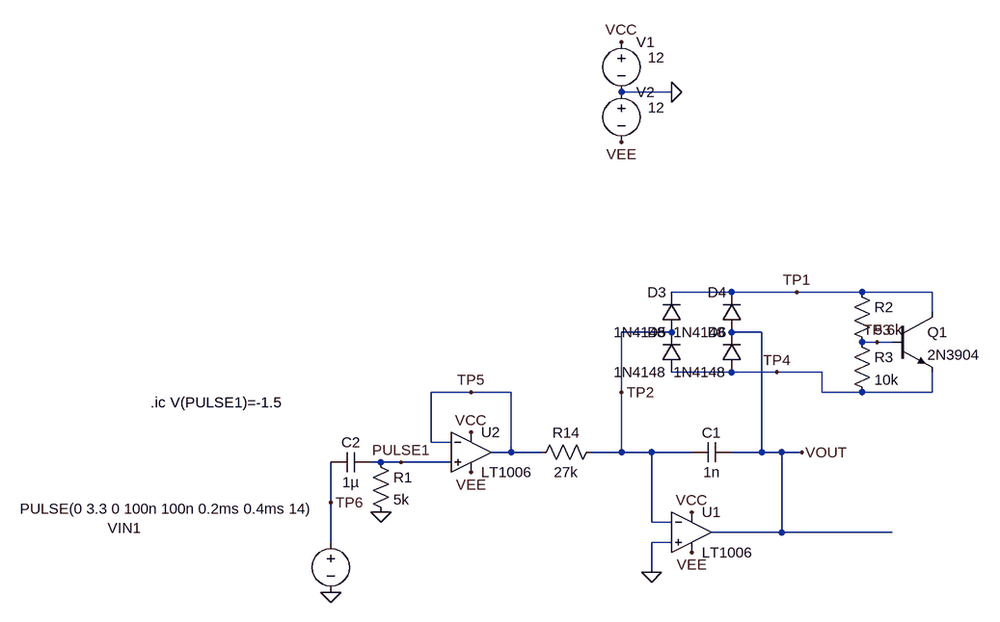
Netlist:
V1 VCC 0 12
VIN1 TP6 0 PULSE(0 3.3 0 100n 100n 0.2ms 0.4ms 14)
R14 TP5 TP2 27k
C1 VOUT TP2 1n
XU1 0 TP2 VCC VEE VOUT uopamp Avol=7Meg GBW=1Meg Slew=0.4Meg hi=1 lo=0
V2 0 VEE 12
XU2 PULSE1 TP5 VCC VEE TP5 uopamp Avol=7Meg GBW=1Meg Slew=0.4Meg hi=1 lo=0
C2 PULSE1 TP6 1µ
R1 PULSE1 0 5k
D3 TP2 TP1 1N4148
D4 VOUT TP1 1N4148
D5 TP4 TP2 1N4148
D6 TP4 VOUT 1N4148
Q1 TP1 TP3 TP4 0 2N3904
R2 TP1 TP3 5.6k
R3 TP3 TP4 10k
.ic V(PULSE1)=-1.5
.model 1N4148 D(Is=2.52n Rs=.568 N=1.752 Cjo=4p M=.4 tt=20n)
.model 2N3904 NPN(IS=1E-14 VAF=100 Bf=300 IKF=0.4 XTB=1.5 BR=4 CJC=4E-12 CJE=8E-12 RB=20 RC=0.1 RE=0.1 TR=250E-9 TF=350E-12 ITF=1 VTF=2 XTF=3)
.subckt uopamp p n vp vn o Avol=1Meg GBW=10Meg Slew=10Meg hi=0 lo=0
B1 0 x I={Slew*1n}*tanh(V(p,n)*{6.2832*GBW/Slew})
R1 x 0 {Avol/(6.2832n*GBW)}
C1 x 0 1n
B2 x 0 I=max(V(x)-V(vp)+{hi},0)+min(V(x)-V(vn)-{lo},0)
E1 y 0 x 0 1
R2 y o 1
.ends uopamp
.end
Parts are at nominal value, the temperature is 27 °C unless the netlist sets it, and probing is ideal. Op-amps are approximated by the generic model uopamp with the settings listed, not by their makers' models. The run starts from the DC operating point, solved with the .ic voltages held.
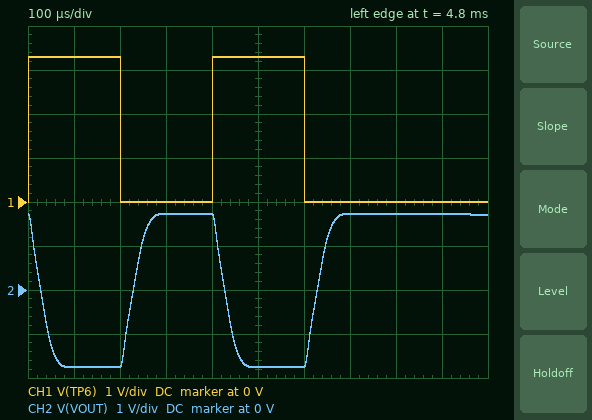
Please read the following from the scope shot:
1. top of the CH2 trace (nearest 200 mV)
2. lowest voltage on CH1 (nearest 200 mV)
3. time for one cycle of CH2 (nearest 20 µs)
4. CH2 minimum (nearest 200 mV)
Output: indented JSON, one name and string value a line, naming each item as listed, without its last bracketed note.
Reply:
{
  "top of the CH2 trace": "1.8 V",
  "lowest voltage on CH1": "0 V",
  "time for one cycle of CH2": "400 µs",
  "CH2 minimum": "-1.8 V"
}
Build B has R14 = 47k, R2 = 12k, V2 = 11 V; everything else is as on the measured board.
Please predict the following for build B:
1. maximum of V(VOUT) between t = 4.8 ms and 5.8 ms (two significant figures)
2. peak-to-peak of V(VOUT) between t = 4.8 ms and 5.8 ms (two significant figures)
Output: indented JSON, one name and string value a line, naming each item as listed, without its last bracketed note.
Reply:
{
  "maximum of V(VOUT) between t = 4.8 ms and 5.8 ms": "1.6 V",
  "peak-to-peak of V(VOUT) between t = 4.8 ms and 5.8 ms": "3.2 V"
}
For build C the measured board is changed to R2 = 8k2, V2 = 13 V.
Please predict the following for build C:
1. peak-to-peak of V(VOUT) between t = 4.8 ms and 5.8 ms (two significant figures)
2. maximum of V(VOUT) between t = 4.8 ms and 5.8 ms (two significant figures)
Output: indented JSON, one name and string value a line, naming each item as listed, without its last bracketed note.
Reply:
{
  "peak-to-peak of V(VOUT) between t = 4.8 ms and 5.8 ms": "3.8 V",
  "maximum of V(VOUT) between t = 4.8 ms and 5.8 ms": "1.9 V"
}
